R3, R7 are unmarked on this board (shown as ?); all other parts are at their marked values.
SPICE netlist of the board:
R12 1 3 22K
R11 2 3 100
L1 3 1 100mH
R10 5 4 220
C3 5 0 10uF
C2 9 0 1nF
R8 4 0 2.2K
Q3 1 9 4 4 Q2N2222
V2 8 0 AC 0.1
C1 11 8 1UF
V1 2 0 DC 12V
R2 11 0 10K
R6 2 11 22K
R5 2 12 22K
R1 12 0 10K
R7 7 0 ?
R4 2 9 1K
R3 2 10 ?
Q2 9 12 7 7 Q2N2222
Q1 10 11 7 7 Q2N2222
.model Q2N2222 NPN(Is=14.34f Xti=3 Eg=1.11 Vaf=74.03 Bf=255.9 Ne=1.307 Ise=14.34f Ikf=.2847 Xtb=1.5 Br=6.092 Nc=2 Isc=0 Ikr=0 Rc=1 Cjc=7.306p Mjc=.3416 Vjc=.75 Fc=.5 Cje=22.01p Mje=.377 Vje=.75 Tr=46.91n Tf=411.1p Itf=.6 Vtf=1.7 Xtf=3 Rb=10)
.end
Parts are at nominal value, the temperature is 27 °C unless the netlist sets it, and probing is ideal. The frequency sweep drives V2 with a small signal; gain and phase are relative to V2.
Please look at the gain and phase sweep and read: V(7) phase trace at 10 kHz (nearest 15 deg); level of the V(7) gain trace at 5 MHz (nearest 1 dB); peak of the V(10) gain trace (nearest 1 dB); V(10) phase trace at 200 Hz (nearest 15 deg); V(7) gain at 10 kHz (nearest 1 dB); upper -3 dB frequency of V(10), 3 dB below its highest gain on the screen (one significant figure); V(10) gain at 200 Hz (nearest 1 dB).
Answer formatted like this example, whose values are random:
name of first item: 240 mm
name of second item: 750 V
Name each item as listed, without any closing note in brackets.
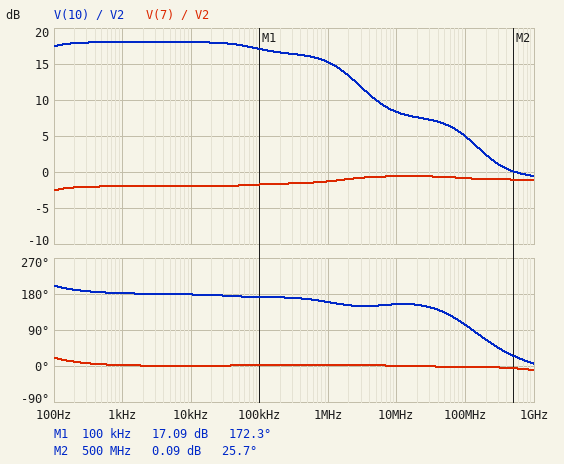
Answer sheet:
V(7) phase trace at 10 kHz: 0 deg
level of the V(7) gain trace at 5 MHz: -1 dB
peak of the V(10) gain trace: 18 dB
V(10) phase trace at 200 Hz: 195 deg
V(7) gain at 10 kHz: -2 dB
upper -3 dB frequency of V(10), 3 dB below its highest gain on the screen: 1 MHz
V(10) gain at 200 Hz: 18 dB
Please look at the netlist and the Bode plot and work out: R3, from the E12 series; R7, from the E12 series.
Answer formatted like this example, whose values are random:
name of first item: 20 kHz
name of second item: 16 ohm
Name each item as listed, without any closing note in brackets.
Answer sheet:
R3, from the E12 series: 470 Ω
R7, from the E12 series: 680 Ω
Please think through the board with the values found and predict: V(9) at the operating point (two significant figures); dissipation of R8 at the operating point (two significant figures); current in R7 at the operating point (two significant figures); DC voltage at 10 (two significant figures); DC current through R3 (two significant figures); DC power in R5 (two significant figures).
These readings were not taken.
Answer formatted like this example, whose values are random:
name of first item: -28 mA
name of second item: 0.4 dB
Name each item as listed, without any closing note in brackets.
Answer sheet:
V(9) at the operating point: 9.8 V
dissipation of R8 at the operating point: 38 mW
current in R7 at the operating point: 4.4 mA
DC voltage at 10: 11 V
DC current through R3: 2.2 mA
DC power in R5: 3.2 mW
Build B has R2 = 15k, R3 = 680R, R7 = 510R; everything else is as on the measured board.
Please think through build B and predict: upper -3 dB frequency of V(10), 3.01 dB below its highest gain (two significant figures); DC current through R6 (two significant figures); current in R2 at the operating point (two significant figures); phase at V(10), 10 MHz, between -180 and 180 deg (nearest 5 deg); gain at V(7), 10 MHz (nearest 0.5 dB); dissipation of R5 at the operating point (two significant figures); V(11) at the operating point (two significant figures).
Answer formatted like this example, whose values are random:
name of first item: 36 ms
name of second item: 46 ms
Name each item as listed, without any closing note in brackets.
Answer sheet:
upper -3 dB frequency of V(10), 3.01 dB below its highest gain: 83 MHz
DC current through R6: 340 µA
current in R2 at the operating point: 300 µA
phase at V(10), 10 MHz, between -180 and 180 deg: 165 deg
gain at V(7), 10 MHz: 0 dB
dissipation of R5 at the operating point: 3.1 mW
V(11) at the operating point: 4.5 V
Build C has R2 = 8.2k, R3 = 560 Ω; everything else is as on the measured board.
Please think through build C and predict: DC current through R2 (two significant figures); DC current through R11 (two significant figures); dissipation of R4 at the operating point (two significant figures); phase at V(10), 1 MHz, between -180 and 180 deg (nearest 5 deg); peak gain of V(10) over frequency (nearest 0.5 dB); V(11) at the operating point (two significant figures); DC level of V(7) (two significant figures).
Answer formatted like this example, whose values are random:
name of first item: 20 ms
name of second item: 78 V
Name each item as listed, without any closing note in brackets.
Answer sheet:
DC current through R2: 400 µA
DC current through R11: 3.2 mA
dissipation of R4 at the operating point: 18 mW
phase at V(10), 1 MHz, between -180 and 180 deg: 90 deg
peak gain of V(10) over frequency: -1.0 dB
V(11) at the operating point: 3.3 V
DC level of V(7): 2.9 V
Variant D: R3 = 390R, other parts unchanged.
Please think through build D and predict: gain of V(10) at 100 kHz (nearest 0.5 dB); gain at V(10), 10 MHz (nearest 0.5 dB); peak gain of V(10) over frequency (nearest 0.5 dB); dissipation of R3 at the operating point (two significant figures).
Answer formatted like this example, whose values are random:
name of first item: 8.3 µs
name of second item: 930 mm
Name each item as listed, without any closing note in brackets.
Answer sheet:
gain of V(10) at 100 kHz: 15.5 dB
gain at V(10), 10 MHz: 6.5 dB
peak gain of V(10) over frequency: 16.5 dB
dissipation of R3 at the operating point: 1.9 mW
